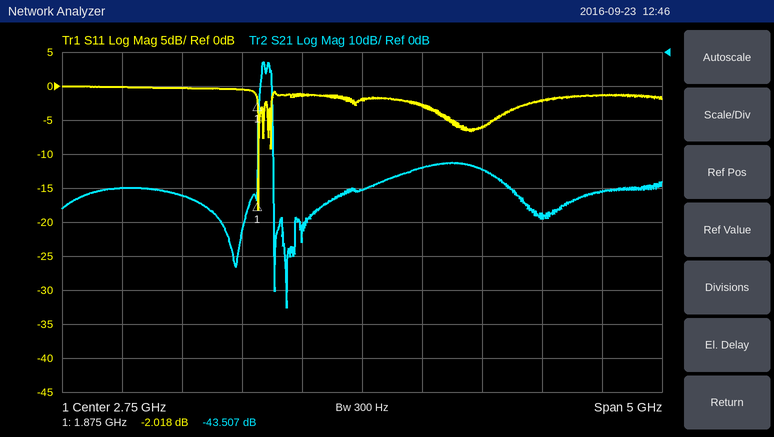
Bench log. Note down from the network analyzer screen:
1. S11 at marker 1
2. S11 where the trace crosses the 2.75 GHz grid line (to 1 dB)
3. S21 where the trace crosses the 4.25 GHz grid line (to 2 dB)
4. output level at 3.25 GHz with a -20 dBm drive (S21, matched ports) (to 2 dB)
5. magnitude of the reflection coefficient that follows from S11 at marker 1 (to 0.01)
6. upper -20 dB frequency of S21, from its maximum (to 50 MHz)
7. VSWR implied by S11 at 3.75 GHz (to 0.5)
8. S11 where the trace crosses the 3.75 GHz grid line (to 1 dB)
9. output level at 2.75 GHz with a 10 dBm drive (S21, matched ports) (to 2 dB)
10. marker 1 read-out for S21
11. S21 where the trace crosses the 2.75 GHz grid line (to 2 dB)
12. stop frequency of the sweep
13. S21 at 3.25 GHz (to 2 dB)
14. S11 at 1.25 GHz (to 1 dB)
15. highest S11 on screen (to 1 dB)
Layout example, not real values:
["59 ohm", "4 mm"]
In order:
["-2.018 dB", "-2 dB", "-48 dB", "-54 dBm", "0.79", "2.00 GHz", "3.0", "-6 dB", "-30 dBm", "-43.507 dB", "-40 dB", "5.25 GHz", "-34 dB", "0 dB", "0 dB"]
